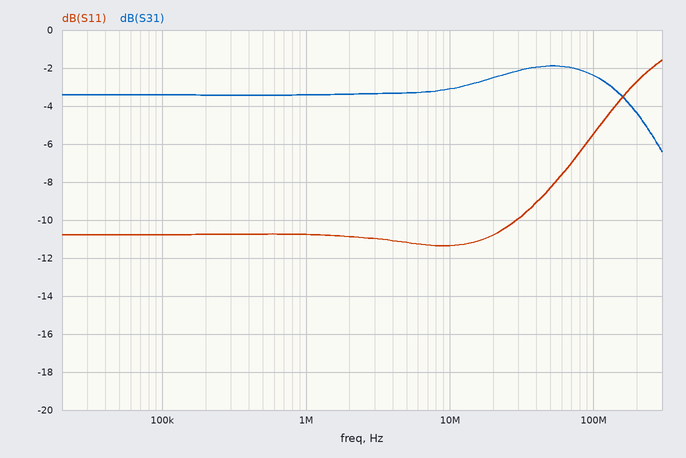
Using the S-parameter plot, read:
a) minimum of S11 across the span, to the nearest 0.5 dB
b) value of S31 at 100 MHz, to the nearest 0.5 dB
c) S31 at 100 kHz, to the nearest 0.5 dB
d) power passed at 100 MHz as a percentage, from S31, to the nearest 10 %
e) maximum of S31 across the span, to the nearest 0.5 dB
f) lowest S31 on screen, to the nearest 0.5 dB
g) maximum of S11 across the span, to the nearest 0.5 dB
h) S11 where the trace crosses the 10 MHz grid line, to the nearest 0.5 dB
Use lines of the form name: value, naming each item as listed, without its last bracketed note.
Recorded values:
minimum of S11 across the span, to the nearest 0.5 dB: -11.5 dB
value of S31 at 100 MHz, to the nearest 0.5 dB: -2.5 dB
S31 at 100 kHz, to the nearest 0.5 dB: -3.5 dB
power passed at 100 MHz as a percentage, from S31, to the nearest 10 %: 60 %
maximum of S31 across the span, to the nearest 0.5 dB: -2.0 dB
lowest S31 on screen, to the nearest 0.5 dB: -6.5 dB
maximum of S11 across the span, to the nearest 0.5 dB: -1.5 dB
S11 where the trace crosses the 10 MHz grid line, to the nearest 0.5 dB: -11.5 dB
